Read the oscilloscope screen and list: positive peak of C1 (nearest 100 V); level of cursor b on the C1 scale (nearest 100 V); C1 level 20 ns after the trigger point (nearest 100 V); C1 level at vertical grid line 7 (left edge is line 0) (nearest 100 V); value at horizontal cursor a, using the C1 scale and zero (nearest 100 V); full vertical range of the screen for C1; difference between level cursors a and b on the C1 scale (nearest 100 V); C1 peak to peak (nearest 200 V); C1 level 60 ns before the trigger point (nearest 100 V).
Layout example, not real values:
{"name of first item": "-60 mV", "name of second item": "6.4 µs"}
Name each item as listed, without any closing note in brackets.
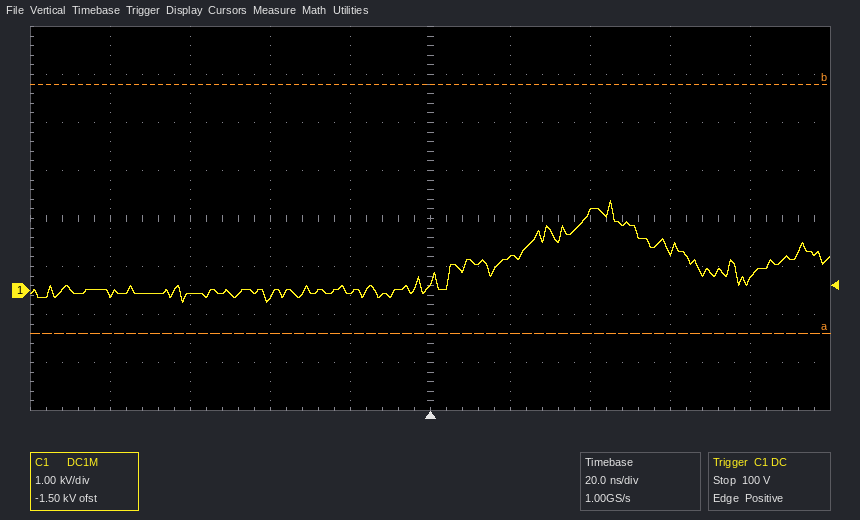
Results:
{"positive peak of C1": "1.9 kV", "level of cursor b on the C1 scale": "4.3 kV", "C1 level 20 ns after the trigger point": "700 V", "C1 level at vertical grid line 7 (left edge is line 0)": "1.6 kV", "value at horizontal cursor a, using the C1 scale and zero": "-900 V", "full vertical range of the screen for C1": "8 kV", "difference between level cursors a and b on the C1 scale": "5.2 kV", "C1 peak to peak": "2.2 kV", "C1 level 60 ns before the trigger point": "-100 V"}
